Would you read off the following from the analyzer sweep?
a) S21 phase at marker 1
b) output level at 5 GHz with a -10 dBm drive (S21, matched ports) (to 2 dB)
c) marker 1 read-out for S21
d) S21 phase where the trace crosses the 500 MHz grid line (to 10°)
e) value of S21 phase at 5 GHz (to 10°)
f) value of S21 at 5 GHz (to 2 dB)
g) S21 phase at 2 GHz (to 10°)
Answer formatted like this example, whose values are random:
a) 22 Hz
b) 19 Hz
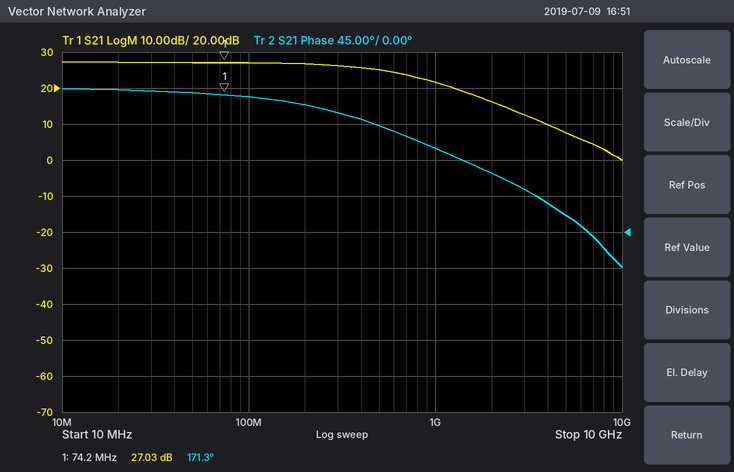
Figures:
a) 171.3°
b) -2 dBm
c) 27.03 dB
d) 130°
e) 20°
f) 8 dB
g) 70°
